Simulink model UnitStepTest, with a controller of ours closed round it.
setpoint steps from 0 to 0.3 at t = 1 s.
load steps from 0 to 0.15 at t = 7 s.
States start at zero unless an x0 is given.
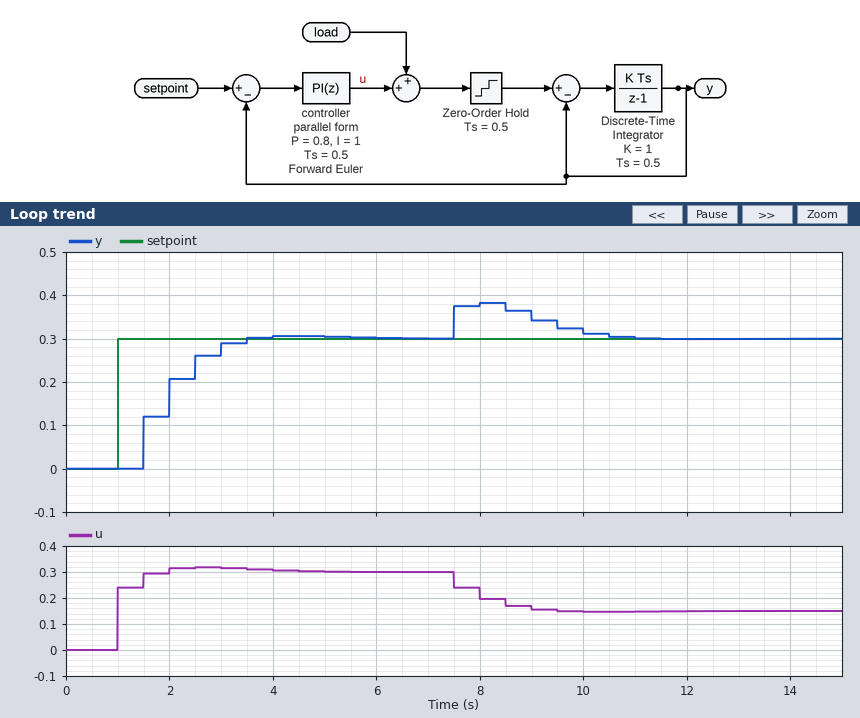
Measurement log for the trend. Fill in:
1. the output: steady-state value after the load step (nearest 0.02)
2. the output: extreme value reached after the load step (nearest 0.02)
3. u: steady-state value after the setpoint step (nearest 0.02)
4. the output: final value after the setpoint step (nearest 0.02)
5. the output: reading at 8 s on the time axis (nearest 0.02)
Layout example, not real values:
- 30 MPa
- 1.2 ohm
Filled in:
- 0.30
- 0.38
- 0.30
- 0.30
- 0.38
